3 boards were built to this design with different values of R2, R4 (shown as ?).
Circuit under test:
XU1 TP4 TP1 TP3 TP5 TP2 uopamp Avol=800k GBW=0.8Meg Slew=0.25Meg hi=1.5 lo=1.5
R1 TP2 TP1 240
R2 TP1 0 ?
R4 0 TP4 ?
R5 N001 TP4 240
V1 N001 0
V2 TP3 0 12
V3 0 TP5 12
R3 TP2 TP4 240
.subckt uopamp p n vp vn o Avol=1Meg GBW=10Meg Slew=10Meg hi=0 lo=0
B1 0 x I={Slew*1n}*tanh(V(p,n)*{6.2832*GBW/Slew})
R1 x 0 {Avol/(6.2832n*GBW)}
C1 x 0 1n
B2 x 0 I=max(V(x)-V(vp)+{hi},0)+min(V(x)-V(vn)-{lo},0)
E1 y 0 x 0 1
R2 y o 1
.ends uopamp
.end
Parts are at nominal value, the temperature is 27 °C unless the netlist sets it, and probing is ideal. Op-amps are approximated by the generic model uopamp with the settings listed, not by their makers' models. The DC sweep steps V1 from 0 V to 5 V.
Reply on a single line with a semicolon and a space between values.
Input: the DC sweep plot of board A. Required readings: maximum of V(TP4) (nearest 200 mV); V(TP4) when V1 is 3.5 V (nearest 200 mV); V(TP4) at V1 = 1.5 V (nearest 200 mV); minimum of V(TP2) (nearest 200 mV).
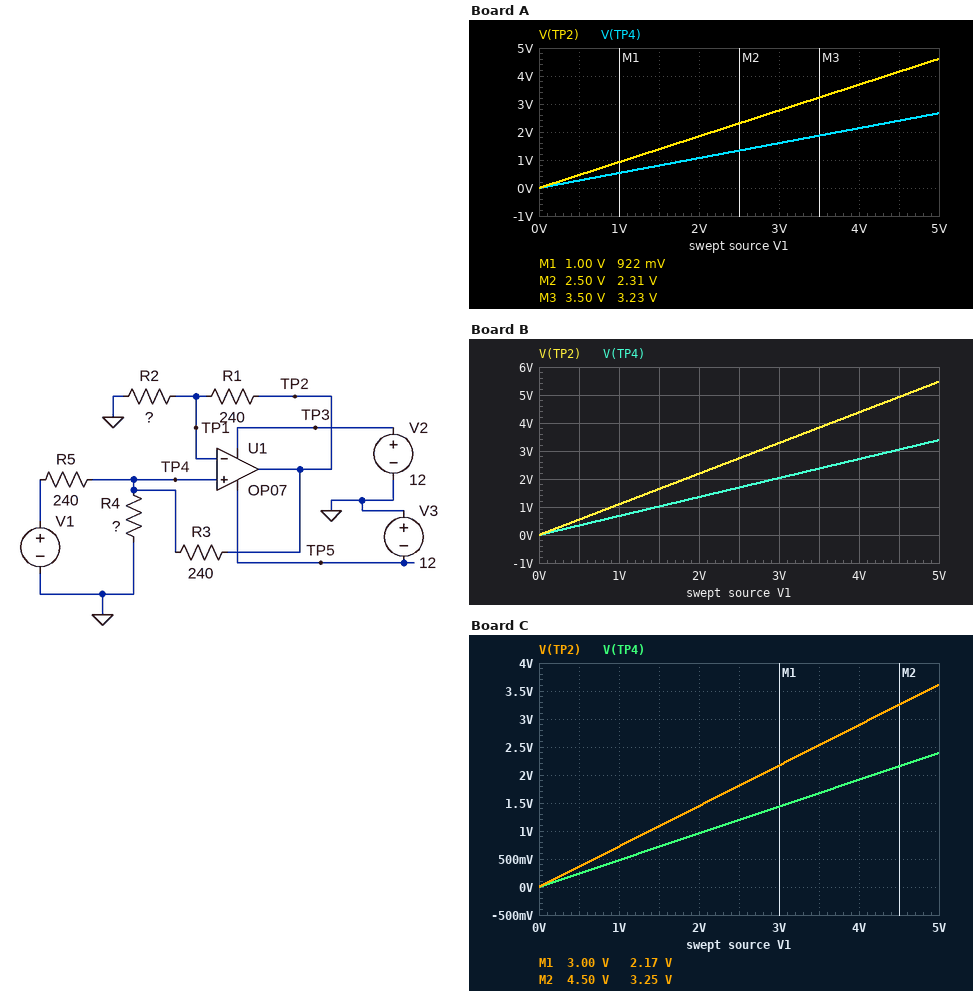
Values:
2.6 V; 1.8 V; 800 mV; 0 V
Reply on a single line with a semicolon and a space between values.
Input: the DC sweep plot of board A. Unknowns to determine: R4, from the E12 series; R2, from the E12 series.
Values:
150 Ω; 330 Ω
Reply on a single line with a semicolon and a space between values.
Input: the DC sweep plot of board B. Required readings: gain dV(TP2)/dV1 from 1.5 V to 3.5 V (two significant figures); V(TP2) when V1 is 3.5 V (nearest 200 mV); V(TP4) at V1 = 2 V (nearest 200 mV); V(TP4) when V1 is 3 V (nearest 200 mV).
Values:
1.1 V/V; 3.8 V; 1.4 V; 2.0 V
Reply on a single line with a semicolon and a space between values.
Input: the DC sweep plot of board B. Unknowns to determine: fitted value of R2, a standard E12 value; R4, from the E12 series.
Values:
390 Ω; 220 Ω
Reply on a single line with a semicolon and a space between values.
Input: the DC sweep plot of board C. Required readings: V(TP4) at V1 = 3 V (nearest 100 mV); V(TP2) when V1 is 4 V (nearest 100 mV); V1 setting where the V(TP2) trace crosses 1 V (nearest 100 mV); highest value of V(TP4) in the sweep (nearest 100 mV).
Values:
1.4 V; 2.9 V; 1.4 V; 2.4 V
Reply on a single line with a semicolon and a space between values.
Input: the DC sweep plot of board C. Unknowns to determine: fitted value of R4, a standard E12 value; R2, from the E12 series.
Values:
150 Ω; 470 Ω
